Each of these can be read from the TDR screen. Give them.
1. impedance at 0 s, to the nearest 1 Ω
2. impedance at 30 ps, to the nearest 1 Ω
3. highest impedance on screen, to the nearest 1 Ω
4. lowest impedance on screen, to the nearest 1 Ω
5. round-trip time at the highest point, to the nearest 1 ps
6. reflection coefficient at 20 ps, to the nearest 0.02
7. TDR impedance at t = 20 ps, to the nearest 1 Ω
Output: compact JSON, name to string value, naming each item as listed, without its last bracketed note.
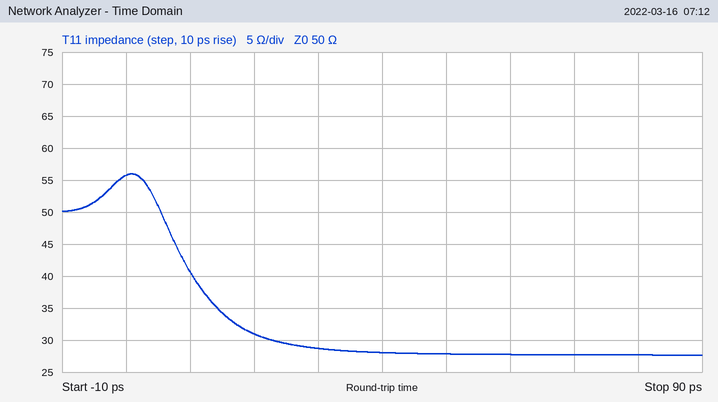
{"impedance at 0 s, to the nearest 1 Ω": "56 Ω", "impedance at 30 ps, to the nearest 1 Ω": "29 Ω", "highest impedance on screen, to the nearest 1 Ω": "56 Ω", "lowest impedance on screen, to the nearest 1 Ω": "28 Ω", "round-trip time at the highest point, to the nearest 1 ps": "1 ps", "reflection coefficient at 20 ps, to the nearest 0.02": "-0.24", "TDR impedance at t = 20 ps, to the nearest 1 Ω": "31 Ω"}
